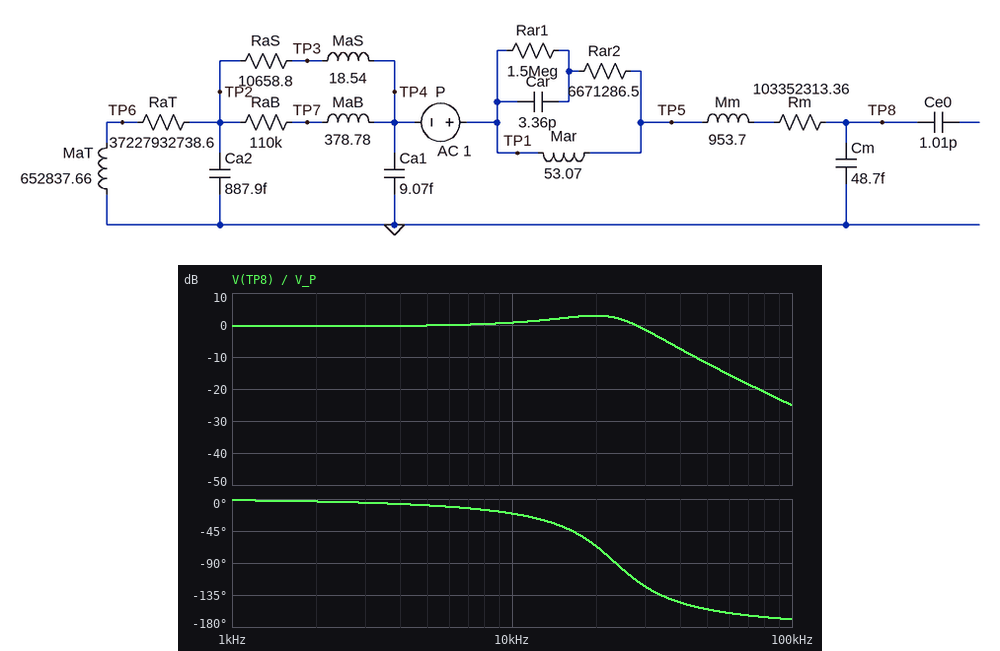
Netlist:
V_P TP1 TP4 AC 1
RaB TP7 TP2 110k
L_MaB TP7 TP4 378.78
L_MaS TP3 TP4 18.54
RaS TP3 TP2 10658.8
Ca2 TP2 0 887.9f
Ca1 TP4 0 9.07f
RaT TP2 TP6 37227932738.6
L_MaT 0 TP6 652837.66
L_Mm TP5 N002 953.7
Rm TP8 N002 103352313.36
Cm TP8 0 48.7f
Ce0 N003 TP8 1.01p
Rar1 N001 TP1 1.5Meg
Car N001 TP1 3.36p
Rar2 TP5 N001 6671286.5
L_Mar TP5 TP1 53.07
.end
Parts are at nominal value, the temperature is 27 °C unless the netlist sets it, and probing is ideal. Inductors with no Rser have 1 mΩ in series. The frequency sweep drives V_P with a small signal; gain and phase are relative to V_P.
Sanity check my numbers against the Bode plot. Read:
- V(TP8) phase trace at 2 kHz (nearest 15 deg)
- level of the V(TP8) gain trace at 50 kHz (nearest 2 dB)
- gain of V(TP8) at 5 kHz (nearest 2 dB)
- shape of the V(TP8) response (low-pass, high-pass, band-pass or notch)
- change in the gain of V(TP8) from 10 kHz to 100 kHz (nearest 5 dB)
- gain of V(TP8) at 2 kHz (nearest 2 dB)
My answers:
0 deg
-12 dB
0 dB
low-pass
-25 dB
0 dB
